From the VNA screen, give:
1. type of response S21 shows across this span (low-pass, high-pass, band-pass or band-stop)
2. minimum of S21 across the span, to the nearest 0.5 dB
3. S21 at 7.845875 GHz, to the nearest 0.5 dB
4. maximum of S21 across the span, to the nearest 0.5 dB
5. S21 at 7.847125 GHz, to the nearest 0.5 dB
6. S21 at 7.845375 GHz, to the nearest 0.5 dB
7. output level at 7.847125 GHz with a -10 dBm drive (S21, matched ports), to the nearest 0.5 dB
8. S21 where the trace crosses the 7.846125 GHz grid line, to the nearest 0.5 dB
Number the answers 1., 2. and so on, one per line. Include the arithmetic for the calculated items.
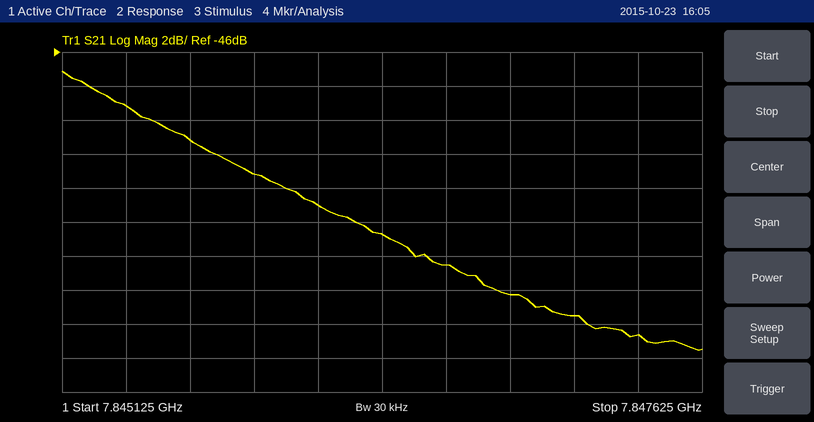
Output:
1. low-pass
2. -63.5 dB
3. -53.0 dB
4. -47.0 dB
5. -61.5 dB
6. -49.0 dB
7. -10 dBm + (-61.5 dB) = -71.5 dBm
8. -55.0 dB
